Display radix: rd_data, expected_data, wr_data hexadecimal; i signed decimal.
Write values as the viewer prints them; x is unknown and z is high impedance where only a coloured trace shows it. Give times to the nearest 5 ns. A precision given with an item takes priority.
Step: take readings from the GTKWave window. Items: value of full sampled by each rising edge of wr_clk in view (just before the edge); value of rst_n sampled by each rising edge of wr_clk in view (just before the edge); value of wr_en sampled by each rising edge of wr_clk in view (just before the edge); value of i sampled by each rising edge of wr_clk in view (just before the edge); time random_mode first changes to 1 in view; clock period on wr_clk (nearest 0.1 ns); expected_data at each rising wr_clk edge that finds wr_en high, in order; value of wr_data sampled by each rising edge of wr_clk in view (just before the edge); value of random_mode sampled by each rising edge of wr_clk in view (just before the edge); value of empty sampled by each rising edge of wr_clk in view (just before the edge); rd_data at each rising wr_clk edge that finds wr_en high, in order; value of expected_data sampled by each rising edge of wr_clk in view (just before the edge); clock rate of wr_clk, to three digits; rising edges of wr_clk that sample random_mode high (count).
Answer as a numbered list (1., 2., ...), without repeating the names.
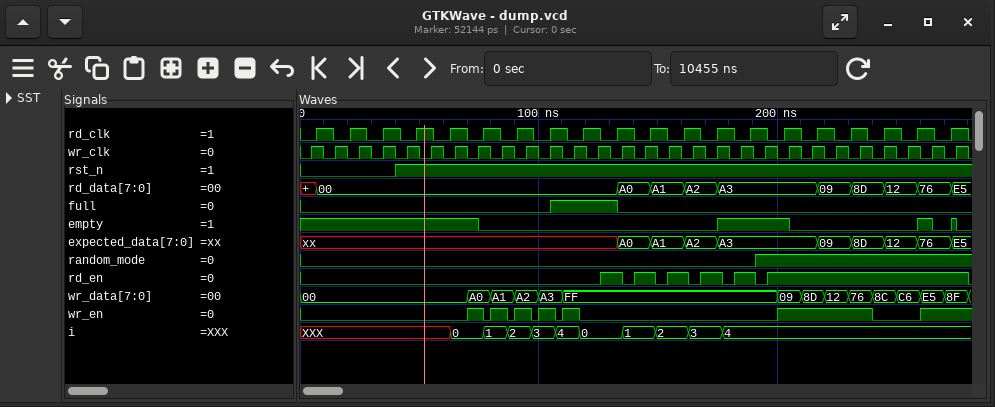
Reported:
1. 0 0 0 0 0 0 0 0 0 0 0 1 1 0 0 0 0 0 0 0 0 0 0 0 0 0 0 0
2. 0 0 0 0 1 1 1 1 1 1 1 1 1 1 1 1 1 1 1 1 1 1 1 1 1 1 1 1
3. 0 0 0 0 0 0 0 1 1 1 1 1 0 0 0 0 0 0 0 0 1 1 1 1 0 0 1 1
4. XXX, XXX, XXX, XXX, XXX, XXX, 0, 0, 1, 2, 3, 4, 0, 0, 1, 2, 3, 3, 4, 4, 4, 4, 4, 4, 4, 4, 4, 4
5. 190 ns
6. 10 ns
7. xx, xx, xx, xx, xx, A3, A3, 09, 8D, 76, E5
8. 00, 00, 00, 00, 00, 00, 00, A0, A1, A2, A3, FF, FF, FF, FF, FF, FF, FF, FF, FF, 09, 8D, 12, 76, 8C, C6, E5, 8F
9. 0 0 0 0 0 0 0 0 0 0 0 0 0 0 0 0 0 0 0 1 1 1 1 1 1 1 1 1
10. 1 1 1 1 1 1 1 1 0 0 0 0 0 0 0 0 0 0 1 1 1 0 0 0 0 0 1 1
11. 00, 00, 00, 00, 00, A3, A3, 09, 8D, 76, E5
12. xx, xx, xx, xx, xx, xx, xx, xx, xx, xx, xx, xx, xx, A0, A0, A1, A2, A2, A3, A3, A3, A3, 09, 8D, 8D, 12, 76, E5
13. 100 MHz
14. 9
